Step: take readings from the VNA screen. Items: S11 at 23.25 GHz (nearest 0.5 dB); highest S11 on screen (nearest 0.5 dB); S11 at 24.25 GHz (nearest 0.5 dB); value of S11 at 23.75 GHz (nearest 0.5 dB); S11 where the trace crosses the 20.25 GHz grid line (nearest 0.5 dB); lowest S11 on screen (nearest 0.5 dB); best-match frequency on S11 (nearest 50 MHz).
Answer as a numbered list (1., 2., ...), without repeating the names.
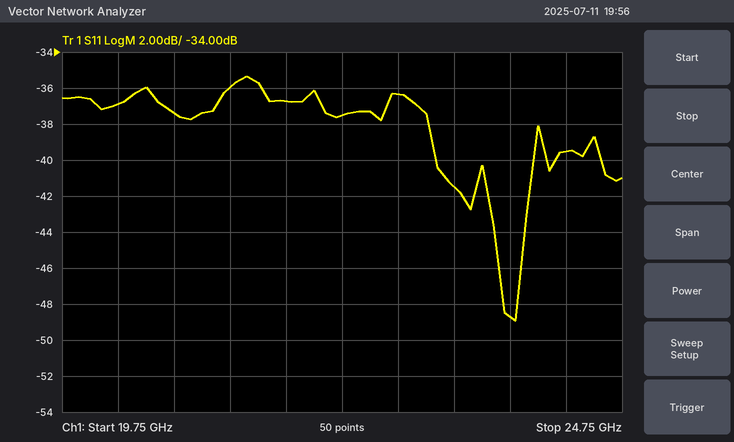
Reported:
1. -41.5 dB
2. -35.5 dB
3. -39.5 dB
4. -48.5 dB
5. -37.0 dB
6. -49.0 dB
7. 23.80 GHz
